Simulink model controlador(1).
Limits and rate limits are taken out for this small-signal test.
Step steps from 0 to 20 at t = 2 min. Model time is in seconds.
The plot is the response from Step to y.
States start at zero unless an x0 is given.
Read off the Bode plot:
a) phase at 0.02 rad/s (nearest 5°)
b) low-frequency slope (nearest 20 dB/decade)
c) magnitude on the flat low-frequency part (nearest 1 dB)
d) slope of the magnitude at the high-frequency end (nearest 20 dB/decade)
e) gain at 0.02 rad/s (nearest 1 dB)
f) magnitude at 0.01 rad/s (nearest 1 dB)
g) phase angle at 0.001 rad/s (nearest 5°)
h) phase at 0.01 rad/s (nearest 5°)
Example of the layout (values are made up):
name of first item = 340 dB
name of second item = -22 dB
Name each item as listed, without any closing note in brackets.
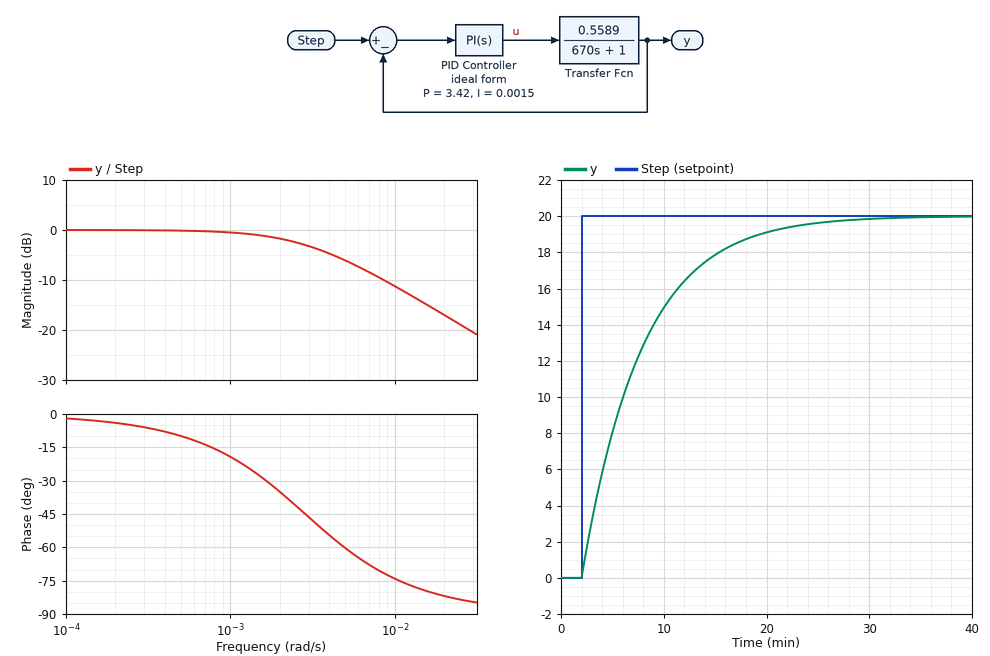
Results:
phase at 0.02 rad/s = -80°
low-frequency slope = 0 dB/decade
magnitude on the flat low-frequency part = 0 dB
slope of the magnitude at the high-frequency end = -20 dB/decade
gain at 0.02 rad/s = -17 dB
magnitude at 0.01 rad/s = -11 dB
phase angle at 0.001 rad/s = -20°
phase at 0.01 rad/s = -75°
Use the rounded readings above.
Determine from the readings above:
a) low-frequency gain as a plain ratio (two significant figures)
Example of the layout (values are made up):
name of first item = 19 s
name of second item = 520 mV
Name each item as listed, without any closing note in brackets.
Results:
low-frequency gain as a plain ratio = 1.0
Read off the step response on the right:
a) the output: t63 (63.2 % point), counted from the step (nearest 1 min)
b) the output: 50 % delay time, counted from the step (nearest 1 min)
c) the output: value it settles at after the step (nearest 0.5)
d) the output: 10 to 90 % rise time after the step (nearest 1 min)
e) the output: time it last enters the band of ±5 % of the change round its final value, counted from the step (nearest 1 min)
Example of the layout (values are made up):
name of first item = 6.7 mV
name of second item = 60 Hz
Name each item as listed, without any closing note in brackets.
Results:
the output: t63 (63.2 % point), counted from the step = 6 min
the output: 50 % delay time, counted from the step = 4 min
the output: value it settles at after the step = 20.0
the output: 10 to 90 % rise time after the step = 13 min
the output: time it last enters the band of ±5 % of the change round its final value, counted from the step = 17 min
